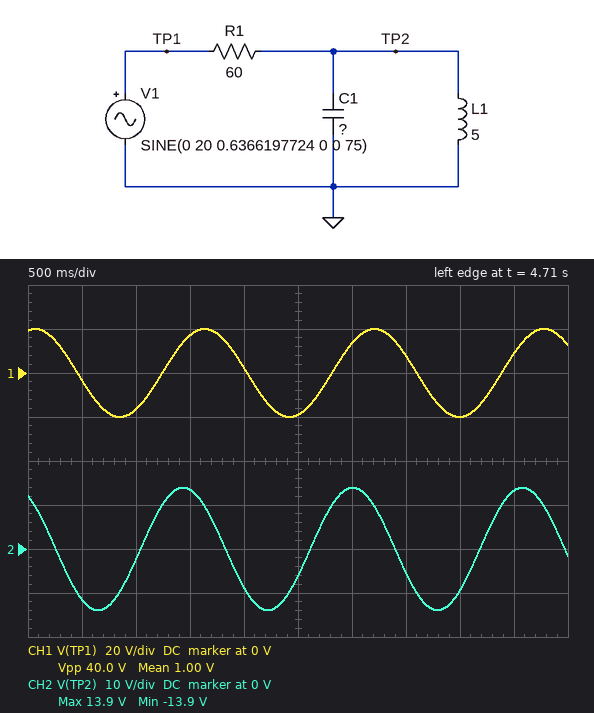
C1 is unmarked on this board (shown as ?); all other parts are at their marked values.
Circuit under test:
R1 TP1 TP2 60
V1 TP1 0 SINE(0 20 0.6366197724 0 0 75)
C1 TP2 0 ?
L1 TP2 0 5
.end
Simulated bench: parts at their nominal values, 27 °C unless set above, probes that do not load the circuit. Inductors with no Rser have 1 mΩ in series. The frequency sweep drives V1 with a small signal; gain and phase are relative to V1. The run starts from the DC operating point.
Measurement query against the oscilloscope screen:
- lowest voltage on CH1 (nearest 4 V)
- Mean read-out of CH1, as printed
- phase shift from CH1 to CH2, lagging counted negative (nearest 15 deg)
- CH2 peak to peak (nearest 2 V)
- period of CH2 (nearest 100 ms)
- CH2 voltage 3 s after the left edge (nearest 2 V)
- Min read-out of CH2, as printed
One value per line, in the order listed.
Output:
-20 V
1.00 V
45 deg
28 V
1.6 s
14 V
-13.9 V
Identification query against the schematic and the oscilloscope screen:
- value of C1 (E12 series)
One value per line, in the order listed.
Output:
8.2 mF
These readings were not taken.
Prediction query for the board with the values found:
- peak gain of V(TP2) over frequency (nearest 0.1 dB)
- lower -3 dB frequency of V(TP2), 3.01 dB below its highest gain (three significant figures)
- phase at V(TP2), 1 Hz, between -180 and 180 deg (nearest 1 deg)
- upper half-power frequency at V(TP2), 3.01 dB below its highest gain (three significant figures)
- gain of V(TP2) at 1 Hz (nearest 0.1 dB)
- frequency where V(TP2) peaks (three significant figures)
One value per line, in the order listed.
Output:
0 dB
641 mHz
-50 deg
964 mHz
-3.8 dB
786 mHz
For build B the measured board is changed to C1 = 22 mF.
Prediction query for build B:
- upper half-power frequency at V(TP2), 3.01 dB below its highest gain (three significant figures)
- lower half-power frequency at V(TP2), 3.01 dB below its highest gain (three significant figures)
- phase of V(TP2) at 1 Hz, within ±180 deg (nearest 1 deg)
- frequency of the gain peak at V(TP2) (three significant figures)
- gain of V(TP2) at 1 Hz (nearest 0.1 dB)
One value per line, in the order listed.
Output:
544 mHz
423 mHz
-81 deg
480 mHz
-16.2 dB
